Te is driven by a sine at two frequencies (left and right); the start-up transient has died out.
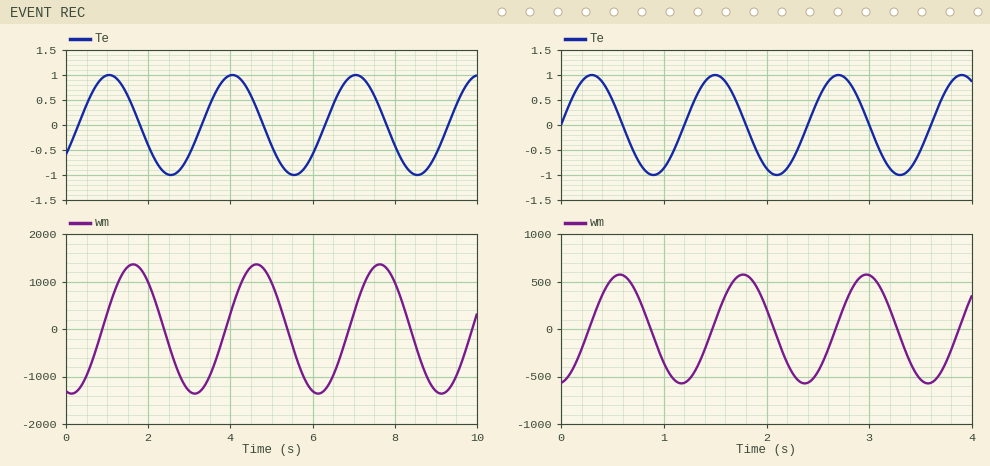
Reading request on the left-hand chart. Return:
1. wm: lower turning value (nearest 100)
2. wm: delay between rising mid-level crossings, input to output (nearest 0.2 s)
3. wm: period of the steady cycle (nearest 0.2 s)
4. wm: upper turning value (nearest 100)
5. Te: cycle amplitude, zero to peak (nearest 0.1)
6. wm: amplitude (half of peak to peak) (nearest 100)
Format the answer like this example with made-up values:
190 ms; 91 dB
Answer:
-1400; 0.6 s; 3.0 s; 1400; 1.0; 1400
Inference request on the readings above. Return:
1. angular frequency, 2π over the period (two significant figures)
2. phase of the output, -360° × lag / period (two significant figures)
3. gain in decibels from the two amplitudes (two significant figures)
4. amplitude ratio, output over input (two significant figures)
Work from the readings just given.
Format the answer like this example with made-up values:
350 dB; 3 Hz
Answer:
2.1 rad/s; -72°; 63 dB; 1400
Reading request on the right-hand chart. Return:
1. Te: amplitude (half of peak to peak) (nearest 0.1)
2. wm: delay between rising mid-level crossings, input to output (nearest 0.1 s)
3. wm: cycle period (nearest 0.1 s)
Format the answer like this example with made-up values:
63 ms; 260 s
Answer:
1.0; 0.3 s; 1.2 s
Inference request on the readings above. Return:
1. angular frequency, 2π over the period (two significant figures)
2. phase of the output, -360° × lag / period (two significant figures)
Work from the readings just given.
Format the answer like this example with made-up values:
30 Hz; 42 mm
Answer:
5.2 rad/s; -90°
